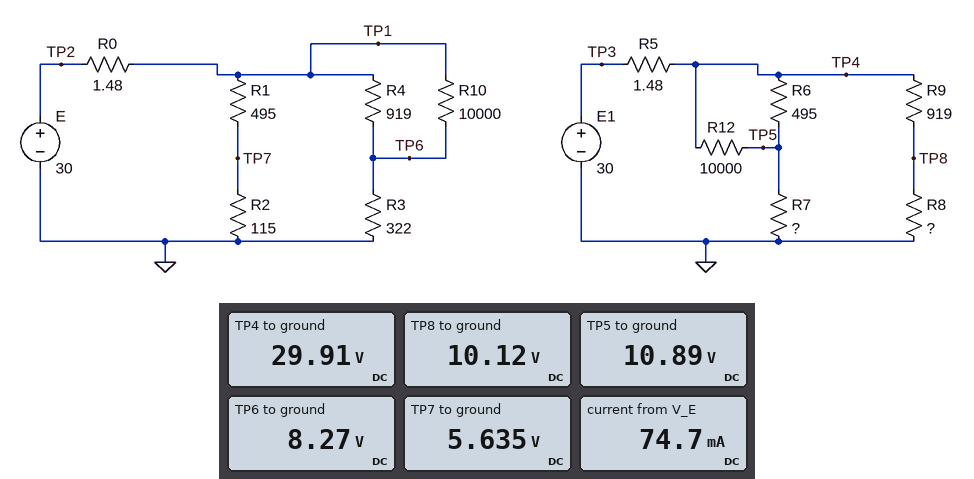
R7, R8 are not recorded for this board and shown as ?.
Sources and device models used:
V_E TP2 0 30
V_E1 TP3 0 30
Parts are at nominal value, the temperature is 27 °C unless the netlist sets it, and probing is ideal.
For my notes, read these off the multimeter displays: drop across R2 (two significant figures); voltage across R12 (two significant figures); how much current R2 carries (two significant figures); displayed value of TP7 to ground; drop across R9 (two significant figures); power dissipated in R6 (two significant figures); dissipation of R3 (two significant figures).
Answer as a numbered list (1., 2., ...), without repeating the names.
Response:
1. 5.6 V
2. 19 V
3. 49 mA
4. 5.635 V
5. 20 V
6. 730 mW
7. 210 mW
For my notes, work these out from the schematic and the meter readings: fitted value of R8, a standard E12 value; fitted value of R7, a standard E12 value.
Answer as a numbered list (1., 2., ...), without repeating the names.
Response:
1. 470 Ω
2. 270 Ω
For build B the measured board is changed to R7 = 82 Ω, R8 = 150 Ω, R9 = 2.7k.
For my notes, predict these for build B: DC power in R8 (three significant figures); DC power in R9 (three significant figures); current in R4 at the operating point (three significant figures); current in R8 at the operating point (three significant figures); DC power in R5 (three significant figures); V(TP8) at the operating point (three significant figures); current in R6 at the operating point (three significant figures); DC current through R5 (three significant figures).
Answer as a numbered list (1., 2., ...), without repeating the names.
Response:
1. 16.5 mW
2. 297 mW
3. 23.5 mA
4. 10.5 mA
5. 6.16 mW
6. 1.57 V
7. 51.5 mA
8. 64.5 mA
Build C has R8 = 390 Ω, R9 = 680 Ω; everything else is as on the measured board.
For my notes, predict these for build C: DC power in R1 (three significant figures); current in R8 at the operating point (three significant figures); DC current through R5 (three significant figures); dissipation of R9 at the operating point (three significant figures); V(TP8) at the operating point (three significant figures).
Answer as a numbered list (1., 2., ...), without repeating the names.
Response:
1. 1.19 W
2. 27.9 mA
3. 68.3 mA
4. 531 mW
5. 10.9 V
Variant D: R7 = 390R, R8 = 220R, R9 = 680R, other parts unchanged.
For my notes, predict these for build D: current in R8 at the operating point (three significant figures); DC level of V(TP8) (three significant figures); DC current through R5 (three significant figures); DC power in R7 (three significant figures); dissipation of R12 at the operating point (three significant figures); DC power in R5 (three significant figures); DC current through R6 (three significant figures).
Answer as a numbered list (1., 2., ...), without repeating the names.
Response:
1. 33.2 mA
2. 7.31 V
3. 67.9 mA
4. 470 mW
5. 26.8 mW
6. 6.83 mW
7. 33.1 mA
